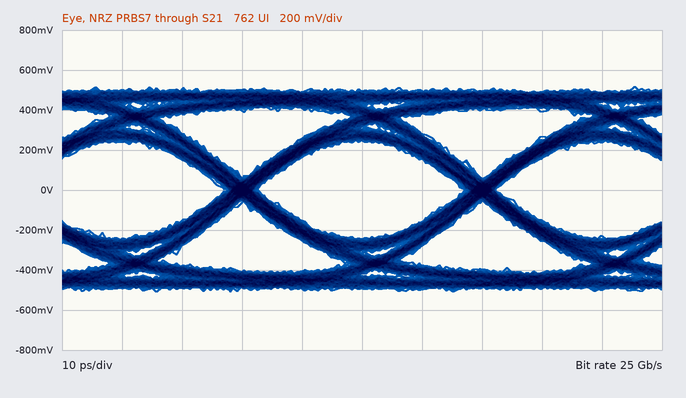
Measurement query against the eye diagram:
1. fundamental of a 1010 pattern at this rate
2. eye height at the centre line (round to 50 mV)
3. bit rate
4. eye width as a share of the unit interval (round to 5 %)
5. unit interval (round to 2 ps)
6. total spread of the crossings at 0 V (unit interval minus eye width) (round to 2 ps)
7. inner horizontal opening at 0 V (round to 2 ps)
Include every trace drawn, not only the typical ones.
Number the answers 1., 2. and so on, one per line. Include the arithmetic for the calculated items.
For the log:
1. 12.5 GHz
2. 500 mV
3. 25 Gb/s
4. 34 ps / 40 ps ≈ 85 %
5. 40 ps
6. 6 ps
7. 34 ps
